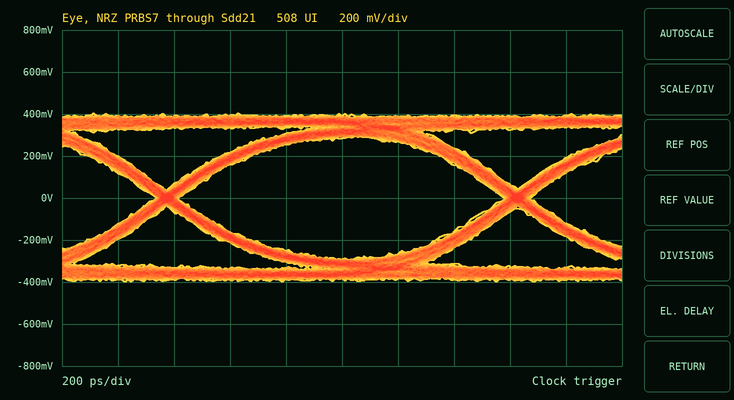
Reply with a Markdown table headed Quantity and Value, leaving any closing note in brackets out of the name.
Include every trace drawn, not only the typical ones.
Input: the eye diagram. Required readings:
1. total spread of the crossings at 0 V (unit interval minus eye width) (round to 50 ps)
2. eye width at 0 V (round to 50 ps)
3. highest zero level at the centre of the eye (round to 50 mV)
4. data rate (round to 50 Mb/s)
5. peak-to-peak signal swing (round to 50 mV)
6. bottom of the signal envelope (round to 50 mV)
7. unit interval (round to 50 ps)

| Quantity | Value |
|---|---|
| total spread of the crossings at 0 V (unit interval minus eye width) | 100 ps |
| eye width at 0 V | 1.15 ns |
| highest zero level at the centre of the eye | -300 mV |
| data rate | 800 Mb/s |
| peak-to-peak signal swing | 800 mV |
| bottom of the signal envelope | -400 mV |
| unit interval | 1.25 ns |
